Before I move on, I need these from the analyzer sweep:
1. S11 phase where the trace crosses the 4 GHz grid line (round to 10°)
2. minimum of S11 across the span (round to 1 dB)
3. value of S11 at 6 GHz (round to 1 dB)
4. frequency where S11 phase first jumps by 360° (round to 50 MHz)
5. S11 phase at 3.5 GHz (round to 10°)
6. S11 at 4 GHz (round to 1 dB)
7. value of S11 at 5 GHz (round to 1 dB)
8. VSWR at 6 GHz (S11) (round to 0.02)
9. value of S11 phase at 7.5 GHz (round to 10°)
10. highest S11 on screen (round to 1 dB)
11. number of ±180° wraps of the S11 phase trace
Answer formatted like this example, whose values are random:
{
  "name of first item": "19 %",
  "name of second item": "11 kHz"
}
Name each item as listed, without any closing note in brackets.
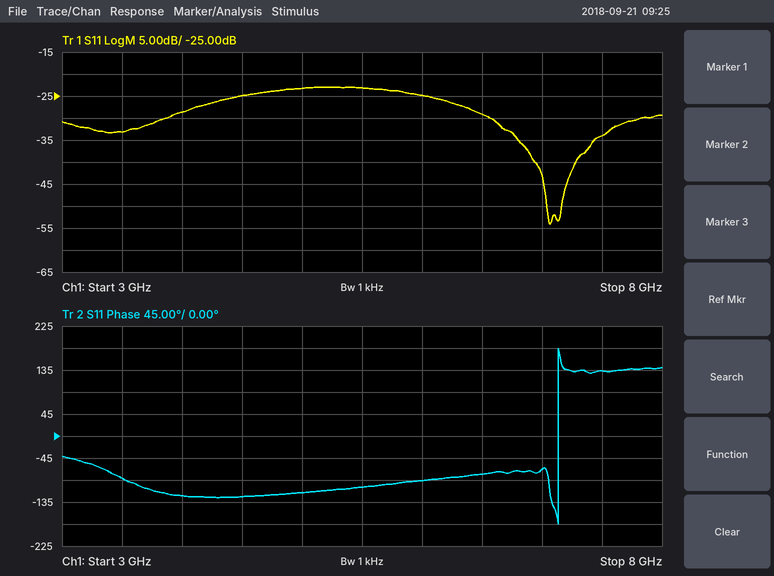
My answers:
{
  "S11 phase where the trace crosses the 4 GHz grid line": "-120°",
  "minimum of S11 across the span": "-54 dB",
  "value of S11 at 6 GHz": "-25 dB",
  "frequency where S11 phase first jumps by 360°": "7.15 GHz",
  "S11 phase at 3.5 GHz": "-90°",
  "S11 at 4 GHz": "-29 dB",
  "value of S11 at 5 GHz": "-23 dB",
  "VSWR at 6 GHz (S11)": "1.12",
  "value of S11 phase at 7.5 GHz": "130°",
  "highest S11 on screen": "-23 dB",
  "number of ±180° wraps of the S11 phase trace": "1"
}
